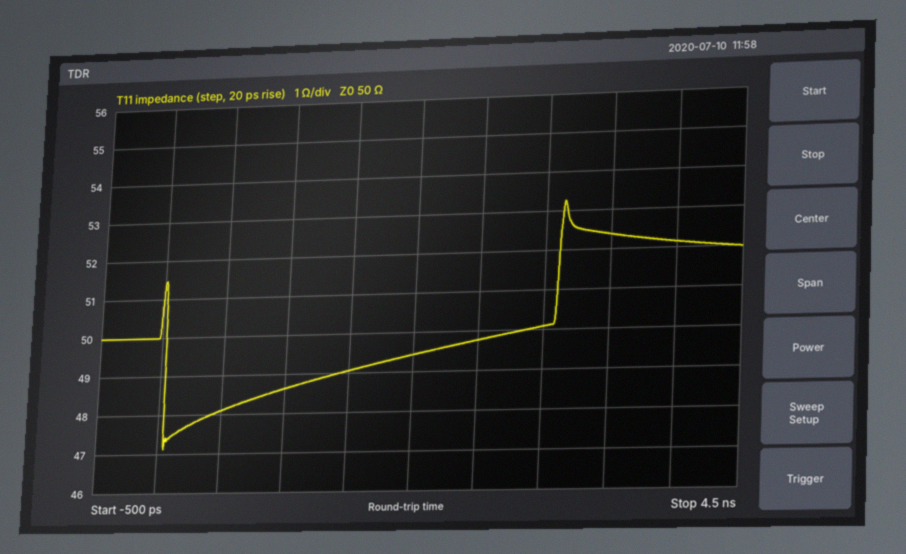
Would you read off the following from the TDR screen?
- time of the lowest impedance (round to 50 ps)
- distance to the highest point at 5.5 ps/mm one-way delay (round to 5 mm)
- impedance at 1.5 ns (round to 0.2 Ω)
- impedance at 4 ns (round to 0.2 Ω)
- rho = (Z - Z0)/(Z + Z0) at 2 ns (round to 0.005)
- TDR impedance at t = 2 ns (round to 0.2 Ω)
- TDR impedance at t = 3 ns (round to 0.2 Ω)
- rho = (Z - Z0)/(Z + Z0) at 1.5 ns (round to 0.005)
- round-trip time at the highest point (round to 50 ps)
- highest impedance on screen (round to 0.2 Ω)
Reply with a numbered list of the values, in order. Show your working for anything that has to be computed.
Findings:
1. 50 ps
2. 3.15 ns / 2 / 5.5 ps/mm ≈ 286 mm, so 285 mm to the nearest 5 mm
3. 49.0 Ω
4. 52.2 Ω
5. (49.4 − 50)/(49.4 + 50) ≈ -0.00604, so -0.005 to the nearest 0.005
6. 49.4 Ω
7. 50.0 Ω
8. (49 − 50)/(49 + 50) ≈ -0.010
9. 3.15 ns
10. 53.2 Ω
